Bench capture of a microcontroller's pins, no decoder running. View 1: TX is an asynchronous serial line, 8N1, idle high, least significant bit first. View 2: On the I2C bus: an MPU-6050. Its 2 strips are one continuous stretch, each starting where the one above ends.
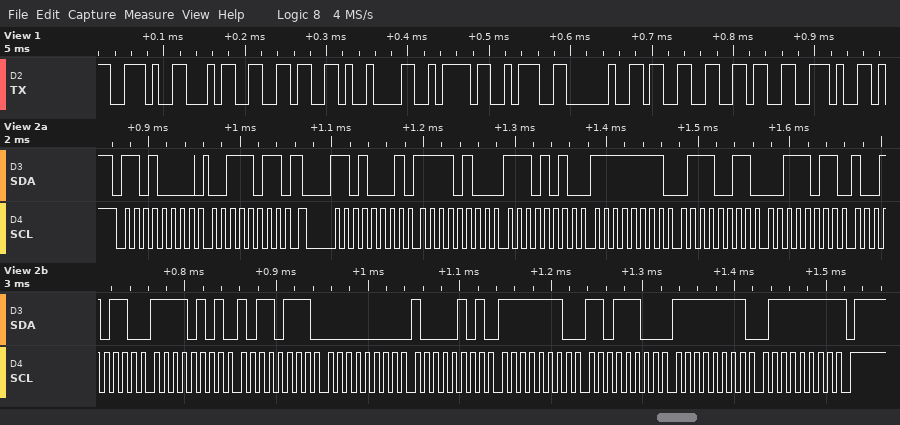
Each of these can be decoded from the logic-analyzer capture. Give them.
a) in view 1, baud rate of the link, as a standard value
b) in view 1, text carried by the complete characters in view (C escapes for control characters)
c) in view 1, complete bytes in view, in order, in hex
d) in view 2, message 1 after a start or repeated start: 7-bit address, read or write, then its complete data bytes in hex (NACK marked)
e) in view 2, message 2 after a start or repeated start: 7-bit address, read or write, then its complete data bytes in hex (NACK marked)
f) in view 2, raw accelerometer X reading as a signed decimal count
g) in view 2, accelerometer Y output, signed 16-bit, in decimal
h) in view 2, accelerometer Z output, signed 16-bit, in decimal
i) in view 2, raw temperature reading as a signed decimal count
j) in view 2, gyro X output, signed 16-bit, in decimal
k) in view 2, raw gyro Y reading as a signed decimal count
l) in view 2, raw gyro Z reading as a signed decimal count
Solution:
115200 baud
".46\tz: 36."
2E 34 36 09 7A 3A 20 33 36 2E
0x68 write: 3B
0x68 read: F4 EA FF 73 3B 96 F5 B7 00 85 FE DC FF 7F NACK
-2838
-141
15254
-2633
133
-292
-129
